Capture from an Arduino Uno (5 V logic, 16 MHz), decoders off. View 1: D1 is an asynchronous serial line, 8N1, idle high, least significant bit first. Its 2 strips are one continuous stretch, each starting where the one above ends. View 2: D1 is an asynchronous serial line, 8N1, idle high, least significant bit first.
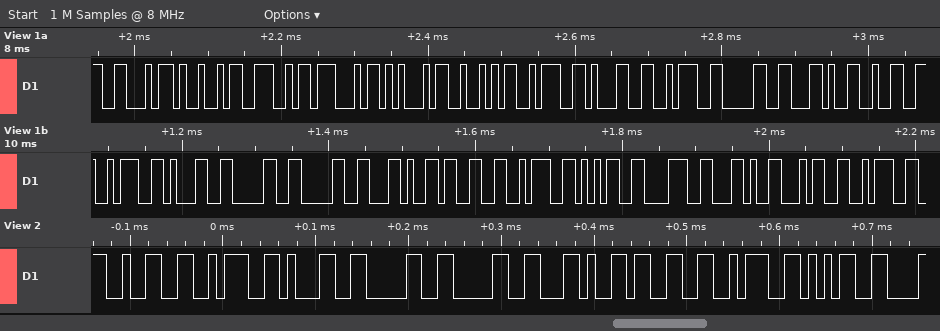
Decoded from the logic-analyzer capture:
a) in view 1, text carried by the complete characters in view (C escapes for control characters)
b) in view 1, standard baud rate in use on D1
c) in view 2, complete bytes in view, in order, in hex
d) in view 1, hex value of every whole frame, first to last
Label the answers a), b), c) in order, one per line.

a) "FINGER:1:0,2:100,3:58,4:"
b) 115200 baud
c) 32 3A 31 30 30 2C 33 3A 35
d) 46 49 4E 47 45 52 3A 31 3A 30 2C 32 3A 31 30 30 2C 33 3A 35 38 2C 34 3A
